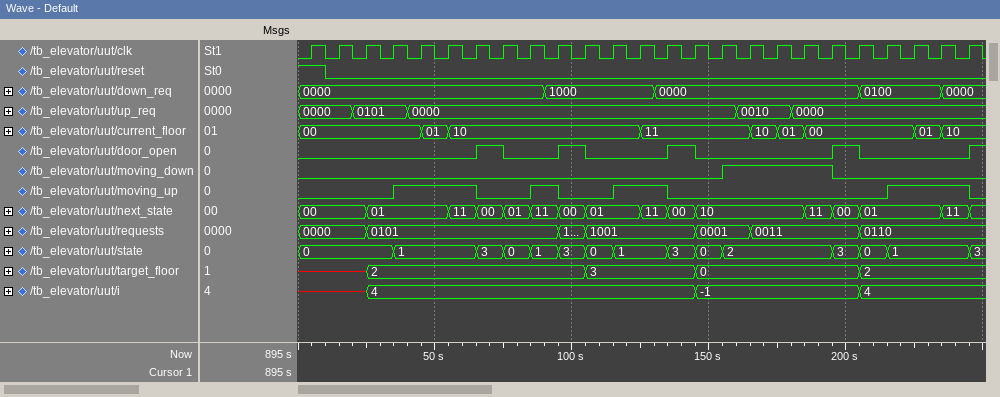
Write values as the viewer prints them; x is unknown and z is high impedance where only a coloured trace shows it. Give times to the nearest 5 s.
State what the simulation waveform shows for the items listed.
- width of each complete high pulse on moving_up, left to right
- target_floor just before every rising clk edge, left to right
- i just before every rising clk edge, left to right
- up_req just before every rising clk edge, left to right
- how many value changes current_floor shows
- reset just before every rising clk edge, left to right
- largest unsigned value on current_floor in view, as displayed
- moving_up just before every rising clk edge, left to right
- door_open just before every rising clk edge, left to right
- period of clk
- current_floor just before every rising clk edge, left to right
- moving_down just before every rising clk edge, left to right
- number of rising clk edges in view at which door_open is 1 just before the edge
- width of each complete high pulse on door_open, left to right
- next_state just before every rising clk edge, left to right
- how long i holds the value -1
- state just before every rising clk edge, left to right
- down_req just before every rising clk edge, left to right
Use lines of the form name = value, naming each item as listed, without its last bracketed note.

width of each complete high pulse on moving_up, left to right = 30 s, 10 s, 20 s, 30 s
target_floor just before every rising clk edge, left to right = x, x, x, 2, 2, 2, 2, 2, 2, 2, 2, 3, 3, 3, 3, 0, 0, 0, 0, 0, 0, 2, 2, 2, 2
i just before every rising clk edge, left to right = x, x, x, 4, 4, 4, 4, 4, 4, 4, 4, 4, 4, 4, 4, -1, -1, -1, -1, -1, -1, 4, 4, 4, 4
up_req just before every rising clk edge, left to right = 0000, 0000, 0101, 0101, 0000, 0000, 0000, 0000, 0000, 0000, 0000, 0000, 0000, 0000, 0000, 0000, 0010, 0010, 0000, 0000, 0000, 0000, 0000, 0000, 0000
how many value changes current_floor shows = 8
reset just before every rising clk edge, left to right = 1 0 0 0 0 0 0 0 0 0 0 0 0 0 0 0 0 0 0 0 0 0 0 0 0
largest unsigned value on current_floor in view, as displayed = 11
moving_up just before every rising clk edge, left to right = 0 0 0 0 1 1 1 0 0 1 0 0 1 1 0 0 0 0 0 0 0 0 1 1 1
door_open just before every rising clk edge, left to right = 0 0 0 0 0 0 0 1 0 0 1 0 0 0 1 0 0 0 0 0 1 0 0 0 0
period of clk = 10 s
current_floor just before every rising clk edge, left to right = 00, 00, 00, 00, 00, 01, 10, 10, 10, 10, 10, 10, 10, 11, 11, 11, 11, 10, 01, 00, 00, 00, 00, 01, 10
moving_down just before every rising clk edge, left to right = 0 0 0 0 0 0 0 0 0 0 0 0 0 0 0 0 1 1 1 1 0 0 0 0 0
number of rising clk edges in view at which door_open is 1 just before the edge = 4
width of each complete high pulse on door_open, left to right = 10 s, 10 s, 10 s, 10 s
next_state just before every rising clk edge, left to right = 00, 00, 00, 01, 01, 01, 11, 00, 01, 11, 00, 01, 01, 11, 00, 10, 10, 10, 10, 11, 00, 01, 01, 01, 11
how long i holds the value -1 = 60 s
state just before every rising clk edge, left to right = 0, 0, 0, 0, 1, 1, 1, 3, 0, 1, 3, 0, 1, 1, 3, 0, 2, 2, 2, 2, 3, 0, 1, 1, 1
down_req just before every rising clk edge, left to right = 0000, 0000, 0000, 0000, 0000, 0000, 0000, 0000, 0000, 1000, 1000, 1000, 1000, 0000, 0000, 0000, 0000, 0000, 0000, 0000, 0000, 0100, 0100, 0100, 0000
